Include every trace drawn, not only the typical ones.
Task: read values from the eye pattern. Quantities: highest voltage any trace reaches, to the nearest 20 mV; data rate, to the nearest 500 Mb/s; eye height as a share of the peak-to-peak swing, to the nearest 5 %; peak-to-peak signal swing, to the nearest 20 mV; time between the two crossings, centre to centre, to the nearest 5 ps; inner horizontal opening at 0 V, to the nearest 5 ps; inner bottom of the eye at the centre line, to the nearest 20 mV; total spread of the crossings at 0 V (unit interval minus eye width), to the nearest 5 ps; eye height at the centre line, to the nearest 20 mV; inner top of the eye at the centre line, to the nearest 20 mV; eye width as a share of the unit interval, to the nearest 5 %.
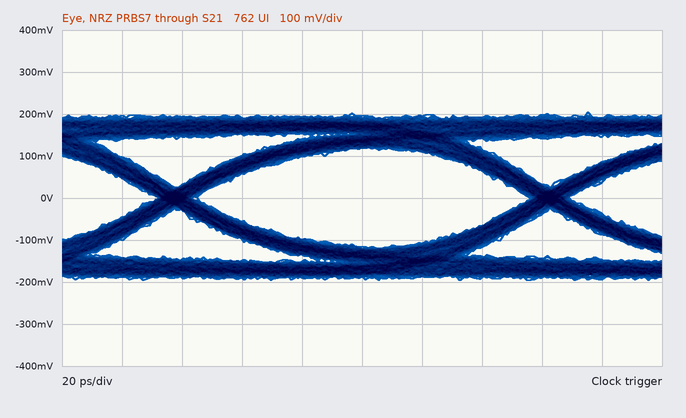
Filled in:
200 mV
8.0 Gb/s
60 %
400 mV
125 ps
110 ps
-120 mV
15 ps
240 mV
120 mV
90 %
